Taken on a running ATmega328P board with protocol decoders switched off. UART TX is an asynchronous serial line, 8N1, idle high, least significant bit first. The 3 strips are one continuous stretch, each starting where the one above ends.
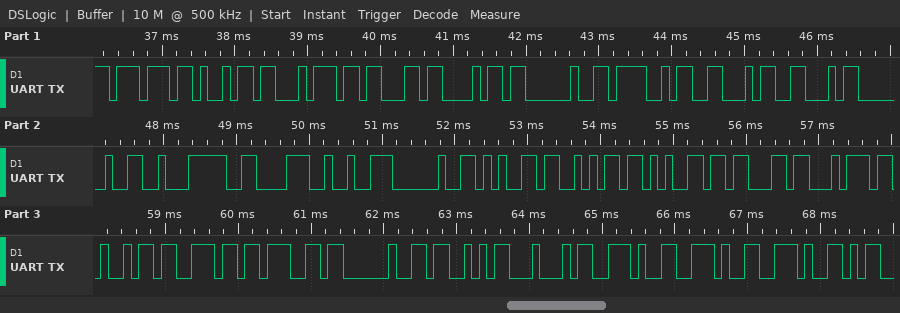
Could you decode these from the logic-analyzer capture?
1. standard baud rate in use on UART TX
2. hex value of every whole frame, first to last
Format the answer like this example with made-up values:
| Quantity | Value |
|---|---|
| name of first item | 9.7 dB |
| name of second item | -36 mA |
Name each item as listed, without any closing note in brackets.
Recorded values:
| Quantity | Value |
|---|---|
| standard baud rate in use on UART TX | 9600 baud |
| hex value of every whole frame, first to last | 77 69 74 63 68 20 4F 46 46 20 E2 86 92 20 65 6A 65 63 74 69 6E 67 20 53 44 2E 2E 2E |
